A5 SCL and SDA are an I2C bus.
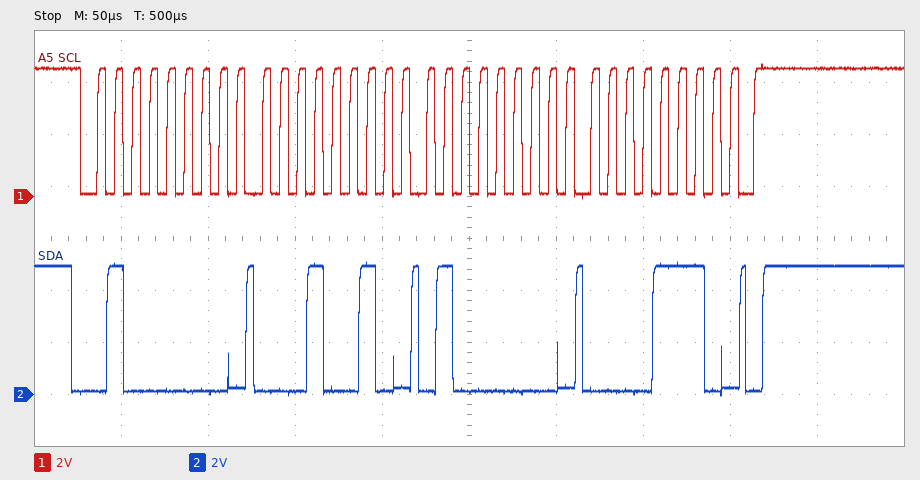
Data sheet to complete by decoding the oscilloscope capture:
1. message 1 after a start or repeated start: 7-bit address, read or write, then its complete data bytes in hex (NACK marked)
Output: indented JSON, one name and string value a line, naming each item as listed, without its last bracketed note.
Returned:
{
  "message 1 after a start or repeated start: 7-bit address, read or write, then its complete data bytes in hex": "0x20 write: 12 40 0E"
}
